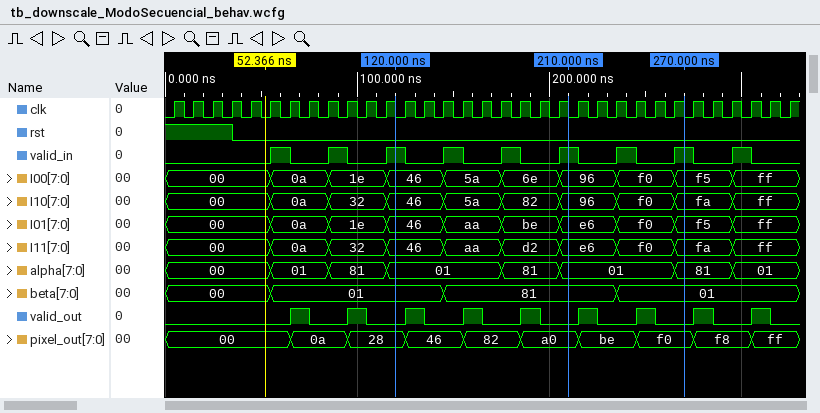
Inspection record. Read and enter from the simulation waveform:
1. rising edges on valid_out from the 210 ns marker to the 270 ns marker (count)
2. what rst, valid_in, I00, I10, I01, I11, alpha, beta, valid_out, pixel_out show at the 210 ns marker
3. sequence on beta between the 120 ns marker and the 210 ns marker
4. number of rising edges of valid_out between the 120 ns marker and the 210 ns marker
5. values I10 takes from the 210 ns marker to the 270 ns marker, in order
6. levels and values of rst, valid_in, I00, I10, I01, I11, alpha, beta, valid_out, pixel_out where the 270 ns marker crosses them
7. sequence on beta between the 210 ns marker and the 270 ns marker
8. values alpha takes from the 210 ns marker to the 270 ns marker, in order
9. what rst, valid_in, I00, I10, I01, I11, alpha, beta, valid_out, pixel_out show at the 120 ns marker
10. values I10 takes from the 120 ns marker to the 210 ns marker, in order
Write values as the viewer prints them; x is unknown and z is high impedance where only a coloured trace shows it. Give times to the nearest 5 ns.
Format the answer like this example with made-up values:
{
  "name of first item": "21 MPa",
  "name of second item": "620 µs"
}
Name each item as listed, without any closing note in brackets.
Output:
{
  "rising edges on valid_out from the 210 ns marker to the 270 ns marker": "2",
  "what rst, valid_in, I00, I10, I01, I11, alpha, beta, valid_out, pixel_out show at the 210 ns marker": "rst=0, valid_in=1, I00=96, I10=96, I01=e6, I11=e6, alpha=01, beta=81, valid_out=0, pixel_out=a0",
  "sequence on beta between the 120 ns marker and the 210 ns marker": "01, 81",
  "number of rising edges of valid_out between the 120 ns marker and the 210 ns marker": "3",
  "values I10 takes from the 210 ns marker to the 270 ns marker, in order": "96, f0, fa",
  "levels and values of rst, valid_in, I00, I10, I01, I11, alpha, beta, valid_out, pixel_out where the 270 ns marker crosses them": "rst=0, valid_in=1, I00=f5, I10=fa, I01=f5, I11=fa, alpha=81, beta=01, valid_out=0, pixel_out=f0",
  "sequence on beta between the 210 ns marker and the 270 ns marker": "81, 01",
  "values alpha takes from the 210 ns marker to the 270 ns marker, in order": "01, 81",
  "what rst, valid_in, I00, I10, I01, I11, alpha, beta, valid_out, pixel_out show at the 120 ns marker": "rst=0, valid_in=1, I00=46, I10=46, I01=46, I11=46, alpha=01, beta=01, valid_out=0, pixel_out=28",
  "values I10 takes from the 120 ns marker to the 210 ns marker, in order": "46, 5a, 82, 96"
}
